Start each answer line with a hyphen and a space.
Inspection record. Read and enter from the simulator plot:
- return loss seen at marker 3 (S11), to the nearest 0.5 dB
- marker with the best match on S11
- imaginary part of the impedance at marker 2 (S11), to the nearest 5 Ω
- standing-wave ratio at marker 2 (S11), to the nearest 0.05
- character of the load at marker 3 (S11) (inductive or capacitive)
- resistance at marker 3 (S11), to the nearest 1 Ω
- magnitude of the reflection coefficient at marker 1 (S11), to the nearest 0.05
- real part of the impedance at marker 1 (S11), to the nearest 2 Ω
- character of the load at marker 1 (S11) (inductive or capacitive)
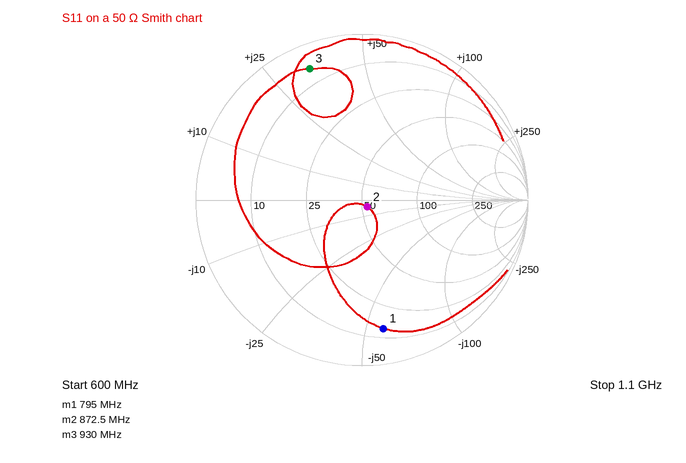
- 1.5 dB
- marker 2
- -5 Ω
- 1.10
- inductive
- 6 Ω
- 0.80
- 14 Ω
- capacitive
